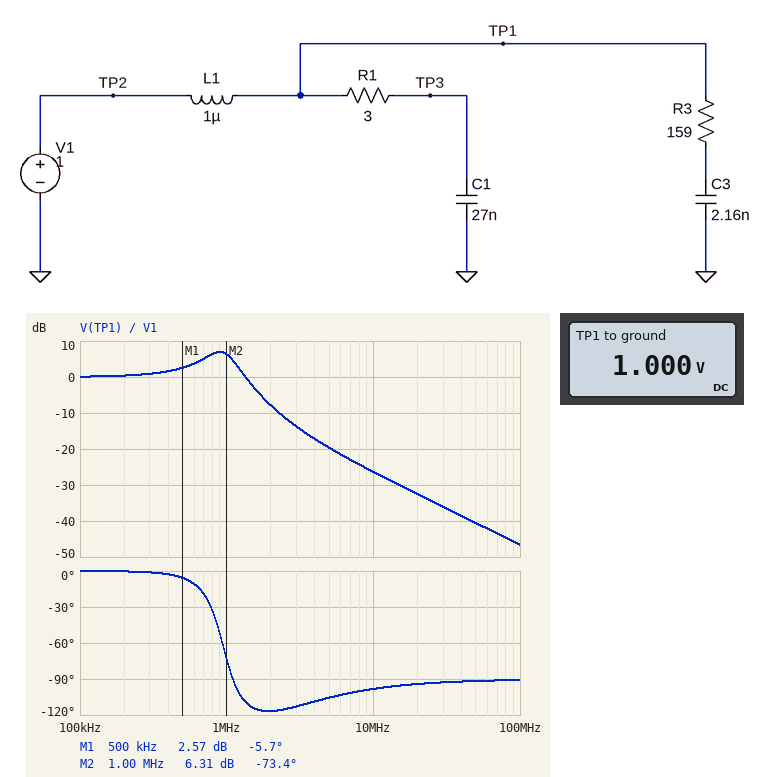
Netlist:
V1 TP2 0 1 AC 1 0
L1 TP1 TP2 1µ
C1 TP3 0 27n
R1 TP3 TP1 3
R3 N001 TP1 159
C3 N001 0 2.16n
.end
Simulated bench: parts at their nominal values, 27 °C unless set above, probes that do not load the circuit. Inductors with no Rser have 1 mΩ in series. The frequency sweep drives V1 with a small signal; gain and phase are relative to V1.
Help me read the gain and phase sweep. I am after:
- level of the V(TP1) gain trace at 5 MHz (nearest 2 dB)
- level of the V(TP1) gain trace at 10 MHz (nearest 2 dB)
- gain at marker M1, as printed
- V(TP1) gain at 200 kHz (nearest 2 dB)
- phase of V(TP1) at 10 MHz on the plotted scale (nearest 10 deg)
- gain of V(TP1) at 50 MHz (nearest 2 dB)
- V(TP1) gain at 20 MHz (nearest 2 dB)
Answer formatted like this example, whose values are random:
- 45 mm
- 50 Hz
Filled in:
- -20 dB
- -26 dB
- 2.57 dB
- 0 dB
- -100 deg
- -40 dB
- -32 dB
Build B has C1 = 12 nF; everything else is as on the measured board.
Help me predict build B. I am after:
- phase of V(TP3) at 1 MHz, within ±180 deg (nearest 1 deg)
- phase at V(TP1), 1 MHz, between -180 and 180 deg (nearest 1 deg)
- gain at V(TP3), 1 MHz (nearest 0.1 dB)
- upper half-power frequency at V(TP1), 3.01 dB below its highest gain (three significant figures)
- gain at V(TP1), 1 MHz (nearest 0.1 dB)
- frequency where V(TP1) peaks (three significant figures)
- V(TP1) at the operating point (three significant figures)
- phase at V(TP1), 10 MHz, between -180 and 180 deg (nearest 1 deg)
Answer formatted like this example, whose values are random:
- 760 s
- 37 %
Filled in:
- -27 deg
- -14 deg
- 5.0 dB
- 1.63 MHz
- 5.2 dB
- 1.38 MHz
- 1.00 V
- -111 deg
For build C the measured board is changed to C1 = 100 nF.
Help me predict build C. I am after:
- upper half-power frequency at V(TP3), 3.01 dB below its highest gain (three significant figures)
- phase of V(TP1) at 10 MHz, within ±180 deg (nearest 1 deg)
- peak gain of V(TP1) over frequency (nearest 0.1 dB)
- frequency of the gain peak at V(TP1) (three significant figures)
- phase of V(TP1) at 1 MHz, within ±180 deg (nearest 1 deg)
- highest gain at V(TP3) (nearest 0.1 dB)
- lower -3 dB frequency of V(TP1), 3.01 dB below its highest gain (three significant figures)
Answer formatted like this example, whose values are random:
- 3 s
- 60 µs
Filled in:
- 587 kHz
- -90 deg
- 3.6 dB
- 431 kHz
- -86 deg
- 1.6 dB
- 131 kHz
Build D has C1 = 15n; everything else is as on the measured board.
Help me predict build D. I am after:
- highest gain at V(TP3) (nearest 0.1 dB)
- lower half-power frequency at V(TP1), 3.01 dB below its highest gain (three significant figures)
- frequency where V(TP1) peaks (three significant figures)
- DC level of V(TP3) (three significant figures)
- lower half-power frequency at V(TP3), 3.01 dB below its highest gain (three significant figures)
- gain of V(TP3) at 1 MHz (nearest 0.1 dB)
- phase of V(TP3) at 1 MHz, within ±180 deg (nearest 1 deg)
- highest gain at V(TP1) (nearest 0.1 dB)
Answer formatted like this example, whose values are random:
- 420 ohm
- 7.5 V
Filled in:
- 8.1 dB
- 938 kHz
- 1.23 MHz
- 1.00 V
- 922 kHz
- 6.1 dB
- -39 deg
- 8.6 dB
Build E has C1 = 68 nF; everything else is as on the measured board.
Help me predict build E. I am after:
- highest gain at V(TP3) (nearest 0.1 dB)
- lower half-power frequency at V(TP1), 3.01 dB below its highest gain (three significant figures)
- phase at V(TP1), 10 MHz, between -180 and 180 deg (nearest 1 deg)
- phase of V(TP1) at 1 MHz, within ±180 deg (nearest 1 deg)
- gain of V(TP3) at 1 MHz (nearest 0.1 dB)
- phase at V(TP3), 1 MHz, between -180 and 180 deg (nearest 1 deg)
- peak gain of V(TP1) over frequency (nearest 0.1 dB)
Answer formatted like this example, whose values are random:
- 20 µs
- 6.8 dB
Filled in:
- 2.9 dB
- 252 kHz
- -92 deg
- -91 deg
- -6.7 dB
- -143 deg
- 4.5 dB
